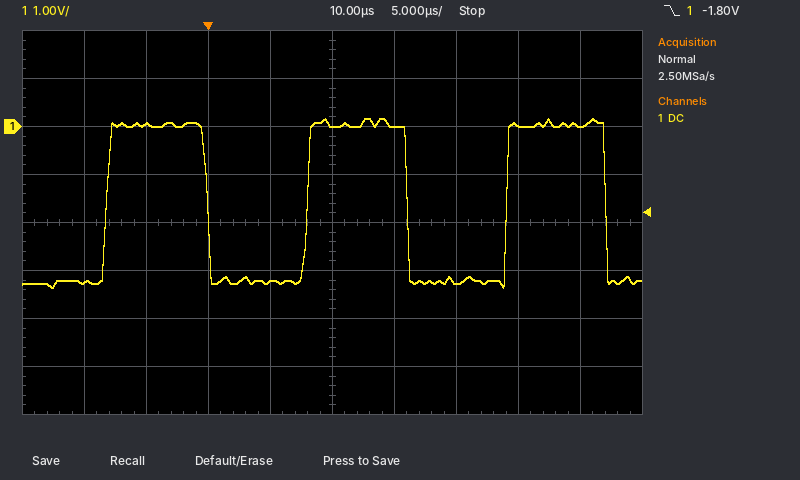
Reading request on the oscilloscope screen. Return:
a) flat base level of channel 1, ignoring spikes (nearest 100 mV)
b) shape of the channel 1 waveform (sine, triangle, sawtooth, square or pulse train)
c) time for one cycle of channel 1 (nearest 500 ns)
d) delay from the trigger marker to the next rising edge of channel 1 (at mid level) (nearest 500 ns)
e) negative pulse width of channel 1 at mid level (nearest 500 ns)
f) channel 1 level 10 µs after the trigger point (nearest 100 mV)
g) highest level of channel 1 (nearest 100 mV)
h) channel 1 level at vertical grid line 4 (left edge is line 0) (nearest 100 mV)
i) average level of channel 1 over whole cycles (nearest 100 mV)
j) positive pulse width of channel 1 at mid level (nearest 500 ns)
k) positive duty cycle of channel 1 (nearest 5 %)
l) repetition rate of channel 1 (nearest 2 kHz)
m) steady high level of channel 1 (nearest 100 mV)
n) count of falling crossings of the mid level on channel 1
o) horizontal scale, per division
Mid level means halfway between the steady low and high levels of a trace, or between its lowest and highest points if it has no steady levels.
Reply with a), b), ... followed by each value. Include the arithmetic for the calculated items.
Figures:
a) -3.2 V
b) square
c) 16.0 µs
d) 8.0 µs
e) 8.0 µs
f) 0.0 V
g) 200 mV
h) -3.2 V
i) -3.2 V + 0.5 × (0.0 V − (-3.2 V)) ≈ -1.6 V
j) 8.0 µs
k) 8.0 µs / 16.0 µs ≈ 50 %
l) 1 / 16.0 µs ≈ 62 kHz
m) 0.0 V
n) 3
o) 5 µs
